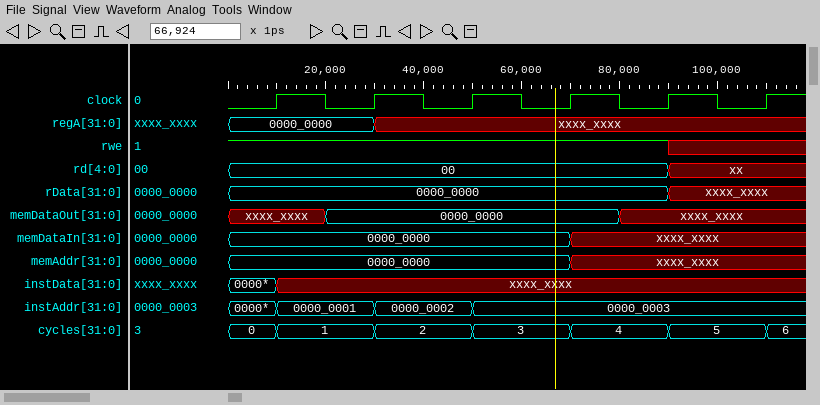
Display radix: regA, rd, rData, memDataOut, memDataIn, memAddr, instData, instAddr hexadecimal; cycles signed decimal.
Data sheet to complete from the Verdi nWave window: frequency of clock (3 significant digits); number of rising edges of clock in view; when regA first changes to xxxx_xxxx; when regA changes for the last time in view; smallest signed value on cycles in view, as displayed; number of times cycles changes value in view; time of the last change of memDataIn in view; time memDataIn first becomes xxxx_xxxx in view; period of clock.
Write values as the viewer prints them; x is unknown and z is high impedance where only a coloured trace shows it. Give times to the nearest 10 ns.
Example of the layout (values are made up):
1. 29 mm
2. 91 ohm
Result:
1. 50.0 MHz
2. 6
3. 30 ns
4. 30 ns
5. 0
6. 6
7. 70 ns
8. 70 ns
9. 20 ns
